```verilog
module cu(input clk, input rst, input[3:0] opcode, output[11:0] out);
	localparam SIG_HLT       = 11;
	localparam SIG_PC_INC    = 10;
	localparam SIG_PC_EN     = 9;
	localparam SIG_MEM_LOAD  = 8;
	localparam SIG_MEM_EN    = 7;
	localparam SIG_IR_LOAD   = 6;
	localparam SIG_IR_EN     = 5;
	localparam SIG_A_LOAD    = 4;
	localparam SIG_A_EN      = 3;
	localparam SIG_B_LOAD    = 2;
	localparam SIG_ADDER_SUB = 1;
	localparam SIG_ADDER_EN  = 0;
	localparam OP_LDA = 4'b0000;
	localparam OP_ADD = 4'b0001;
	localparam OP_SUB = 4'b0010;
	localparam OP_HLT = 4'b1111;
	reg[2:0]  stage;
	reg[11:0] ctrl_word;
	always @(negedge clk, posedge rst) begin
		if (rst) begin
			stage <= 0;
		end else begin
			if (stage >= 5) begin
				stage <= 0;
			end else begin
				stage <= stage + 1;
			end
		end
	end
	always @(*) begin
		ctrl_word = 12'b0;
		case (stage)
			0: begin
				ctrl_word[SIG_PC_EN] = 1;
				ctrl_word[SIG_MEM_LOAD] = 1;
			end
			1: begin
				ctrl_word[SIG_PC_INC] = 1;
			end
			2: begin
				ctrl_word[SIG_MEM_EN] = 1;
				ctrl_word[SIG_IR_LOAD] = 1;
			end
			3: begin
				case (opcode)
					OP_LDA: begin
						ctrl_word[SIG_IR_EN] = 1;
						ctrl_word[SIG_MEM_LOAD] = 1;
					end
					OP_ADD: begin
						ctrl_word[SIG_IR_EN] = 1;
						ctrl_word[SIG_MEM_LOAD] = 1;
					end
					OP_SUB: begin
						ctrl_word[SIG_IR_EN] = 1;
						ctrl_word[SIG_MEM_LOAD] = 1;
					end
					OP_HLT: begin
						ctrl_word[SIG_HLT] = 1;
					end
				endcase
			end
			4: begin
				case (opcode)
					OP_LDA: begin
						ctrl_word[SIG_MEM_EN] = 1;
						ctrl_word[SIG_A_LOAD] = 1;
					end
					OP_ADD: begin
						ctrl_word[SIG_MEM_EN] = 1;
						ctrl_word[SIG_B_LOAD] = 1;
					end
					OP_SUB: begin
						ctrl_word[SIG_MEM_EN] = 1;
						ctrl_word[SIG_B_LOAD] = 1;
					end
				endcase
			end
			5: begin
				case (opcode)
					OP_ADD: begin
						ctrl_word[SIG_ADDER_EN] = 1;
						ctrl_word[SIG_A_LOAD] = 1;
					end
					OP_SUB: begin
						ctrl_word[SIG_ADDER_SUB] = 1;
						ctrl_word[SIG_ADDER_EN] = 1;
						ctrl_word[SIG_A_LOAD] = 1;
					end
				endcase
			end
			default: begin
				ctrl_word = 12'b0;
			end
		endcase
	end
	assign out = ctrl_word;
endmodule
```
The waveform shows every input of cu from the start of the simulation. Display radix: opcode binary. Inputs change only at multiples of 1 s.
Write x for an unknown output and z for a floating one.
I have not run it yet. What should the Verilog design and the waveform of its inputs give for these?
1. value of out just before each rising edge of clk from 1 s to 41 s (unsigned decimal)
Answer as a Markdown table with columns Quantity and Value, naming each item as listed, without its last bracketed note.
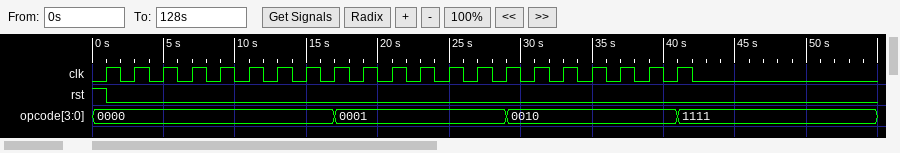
| Quantity | Value |
|---|---|
| value of out just before each rising edge of clk from 1 s to 41 s | 768, 1024, 192, 288, 144, 0, 768, 1024, 192, 288, 132, 17, 768, 1024, 192, 288, 132, 19, 768, 1024, 192 |
